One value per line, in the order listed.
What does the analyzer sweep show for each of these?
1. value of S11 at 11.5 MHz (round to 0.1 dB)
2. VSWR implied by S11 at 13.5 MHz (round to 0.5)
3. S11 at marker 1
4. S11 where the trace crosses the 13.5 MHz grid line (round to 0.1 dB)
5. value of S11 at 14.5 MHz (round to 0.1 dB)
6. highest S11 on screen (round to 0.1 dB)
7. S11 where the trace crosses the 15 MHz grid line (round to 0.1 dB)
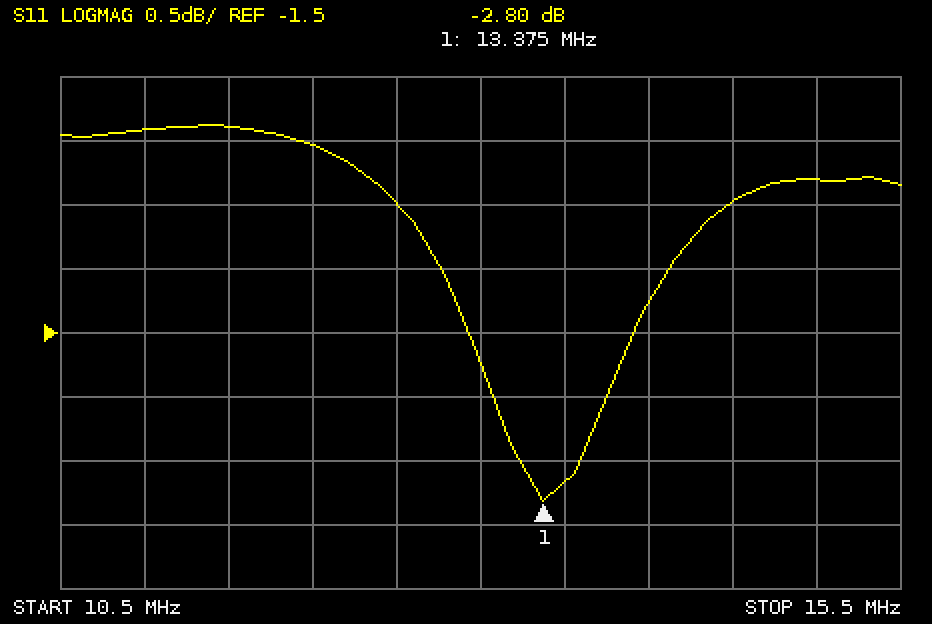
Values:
0.1 dB
6.5
-2.80 dB
-2.7 dB
-0.5 dB
0.1 dB
-0.3 dB
